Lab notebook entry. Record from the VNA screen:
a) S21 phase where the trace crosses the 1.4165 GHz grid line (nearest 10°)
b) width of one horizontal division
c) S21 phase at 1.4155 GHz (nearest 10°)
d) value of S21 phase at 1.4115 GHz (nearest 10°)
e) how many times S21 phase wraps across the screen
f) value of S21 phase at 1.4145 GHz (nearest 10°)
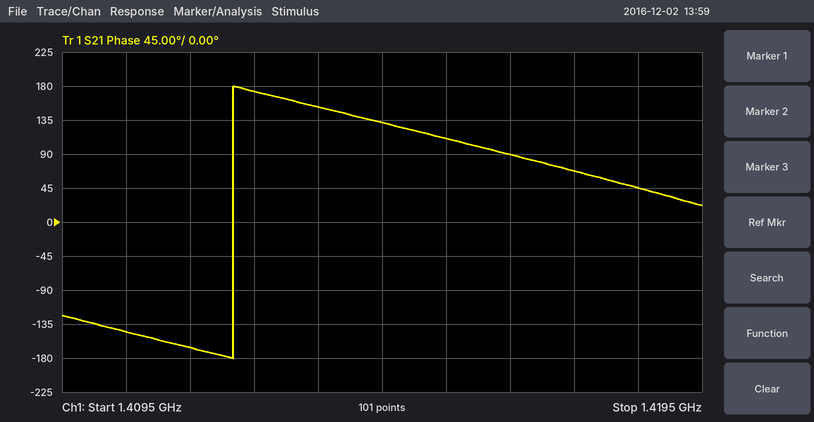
90°
1 MHz
110°
-170°
1
130°
